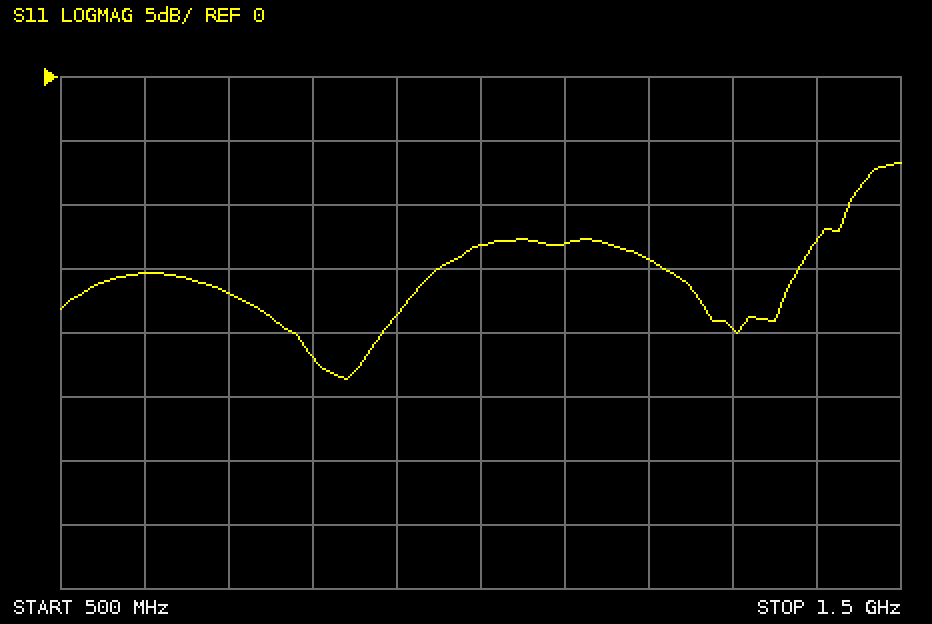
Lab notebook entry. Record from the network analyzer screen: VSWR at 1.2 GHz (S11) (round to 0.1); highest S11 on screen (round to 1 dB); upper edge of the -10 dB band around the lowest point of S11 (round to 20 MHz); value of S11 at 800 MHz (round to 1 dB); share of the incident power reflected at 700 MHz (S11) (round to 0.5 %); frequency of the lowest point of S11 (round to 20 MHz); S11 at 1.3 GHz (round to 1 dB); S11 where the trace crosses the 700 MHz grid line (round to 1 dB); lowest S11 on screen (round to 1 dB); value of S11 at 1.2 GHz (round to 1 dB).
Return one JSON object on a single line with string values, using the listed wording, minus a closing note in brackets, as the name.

{"VSWR at 1.2 GHz (S11)": "1.5", "highest S11 on screen": "-7 dB", "upper edge of the -10 dB band around the lowest point of S11": "1.44 GHz", "value of S11 at 800 MHz": "-22 dB", "share of the incident power reflected at 700 MHz (S11)": "2.0 %", "frequency of the lowest point of S11": "840 MHz", "S11 at 1.3 GHz": "-20 dB", "S11 where the trace crosses the 700 MHz grid line": "-17 dB", "lowest S11 on screen": "-24 dB", "value of S11 at 1.2 GHz": "-14 dB"}
